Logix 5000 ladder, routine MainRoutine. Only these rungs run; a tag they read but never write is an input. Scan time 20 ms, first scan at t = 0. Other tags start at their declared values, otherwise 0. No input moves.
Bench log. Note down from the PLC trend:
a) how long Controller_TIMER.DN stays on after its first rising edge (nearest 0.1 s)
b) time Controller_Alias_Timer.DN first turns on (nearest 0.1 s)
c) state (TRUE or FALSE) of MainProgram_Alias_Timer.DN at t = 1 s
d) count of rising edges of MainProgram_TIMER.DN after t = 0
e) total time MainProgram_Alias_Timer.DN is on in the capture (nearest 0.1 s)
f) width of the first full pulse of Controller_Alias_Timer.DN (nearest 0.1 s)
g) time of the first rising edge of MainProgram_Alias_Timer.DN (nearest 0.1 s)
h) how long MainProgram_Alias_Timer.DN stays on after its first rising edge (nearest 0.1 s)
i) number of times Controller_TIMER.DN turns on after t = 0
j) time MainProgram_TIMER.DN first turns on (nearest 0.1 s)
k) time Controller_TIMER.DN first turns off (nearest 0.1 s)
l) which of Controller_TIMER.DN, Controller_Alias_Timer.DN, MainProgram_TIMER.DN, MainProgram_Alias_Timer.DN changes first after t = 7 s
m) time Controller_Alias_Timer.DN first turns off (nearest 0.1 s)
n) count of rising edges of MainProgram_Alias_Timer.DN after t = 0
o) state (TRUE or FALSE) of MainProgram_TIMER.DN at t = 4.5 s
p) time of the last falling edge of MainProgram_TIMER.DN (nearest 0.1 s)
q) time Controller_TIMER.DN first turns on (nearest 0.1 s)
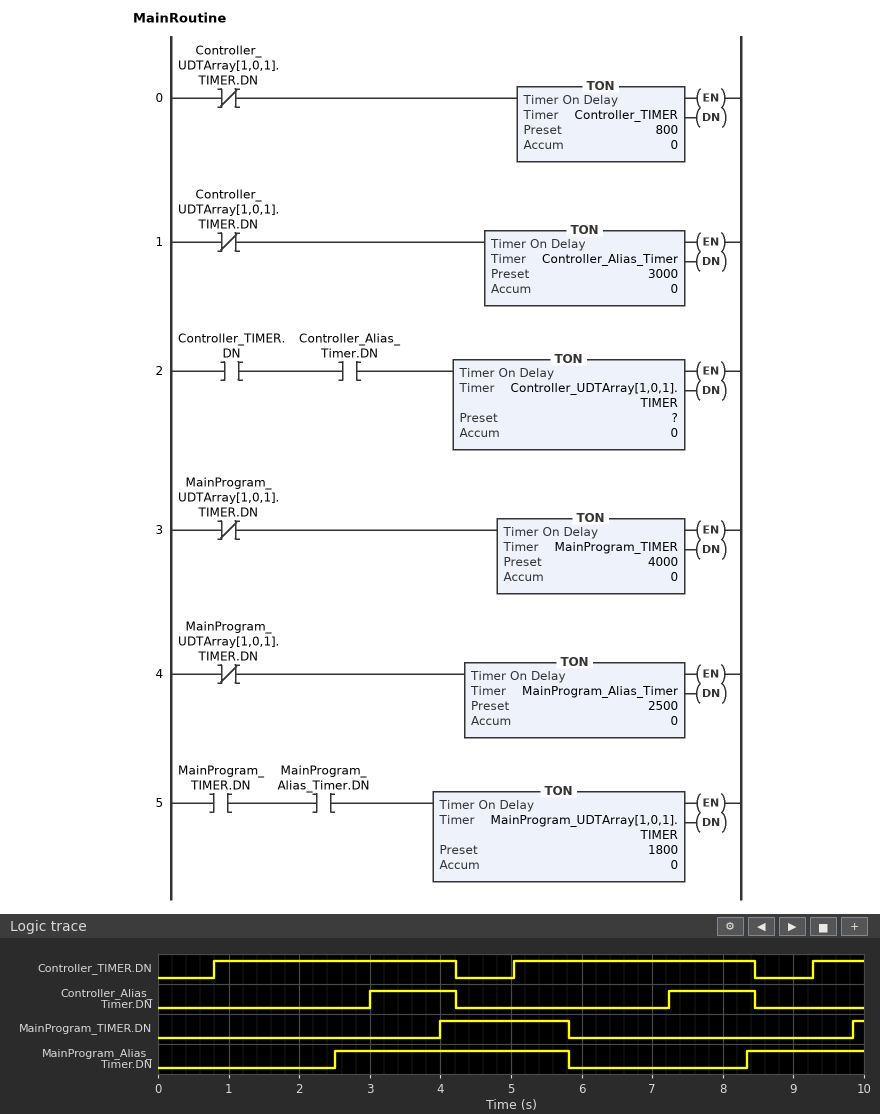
3.4 s
3.0 s
FALSE
2
5.0 s
1.2 s
2.5 s
3.3 s
3
4.0 s
4.2 s
Controller_Alias_Timer.DN
4.2 s
2
TRUE
5.8 s
0.8 s
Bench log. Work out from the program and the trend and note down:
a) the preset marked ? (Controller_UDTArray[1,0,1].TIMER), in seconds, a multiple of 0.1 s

1.2 s
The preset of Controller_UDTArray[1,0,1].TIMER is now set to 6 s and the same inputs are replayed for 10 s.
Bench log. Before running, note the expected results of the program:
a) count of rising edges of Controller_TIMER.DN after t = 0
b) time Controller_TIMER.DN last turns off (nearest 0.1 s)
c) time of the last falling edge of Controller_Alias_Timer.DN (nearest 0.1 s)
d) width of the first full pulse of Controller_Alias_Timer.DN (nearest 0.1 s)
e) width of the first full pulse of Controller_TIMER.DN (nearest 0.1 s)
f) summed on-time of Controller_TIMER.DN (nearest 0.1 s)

2
9.0 s
9.0 s
6.0 s
8.2 s
8.4 s
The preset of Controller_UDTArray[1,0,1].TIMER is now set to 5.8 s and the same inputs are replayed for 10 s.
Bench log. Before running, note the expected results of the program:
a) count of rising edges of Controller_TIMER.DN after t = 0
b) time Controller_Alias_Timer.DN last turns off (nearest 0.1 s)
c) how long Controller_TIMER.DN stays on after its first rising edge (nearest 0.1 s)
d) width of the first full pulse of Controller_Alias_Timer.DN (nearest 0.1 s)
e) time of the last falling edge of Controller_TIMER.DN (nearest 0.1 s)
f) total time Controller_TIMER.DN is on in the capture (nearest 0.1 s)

2
8.8 s
8.0 s
5.8 s
8.8 s
8.4 s
